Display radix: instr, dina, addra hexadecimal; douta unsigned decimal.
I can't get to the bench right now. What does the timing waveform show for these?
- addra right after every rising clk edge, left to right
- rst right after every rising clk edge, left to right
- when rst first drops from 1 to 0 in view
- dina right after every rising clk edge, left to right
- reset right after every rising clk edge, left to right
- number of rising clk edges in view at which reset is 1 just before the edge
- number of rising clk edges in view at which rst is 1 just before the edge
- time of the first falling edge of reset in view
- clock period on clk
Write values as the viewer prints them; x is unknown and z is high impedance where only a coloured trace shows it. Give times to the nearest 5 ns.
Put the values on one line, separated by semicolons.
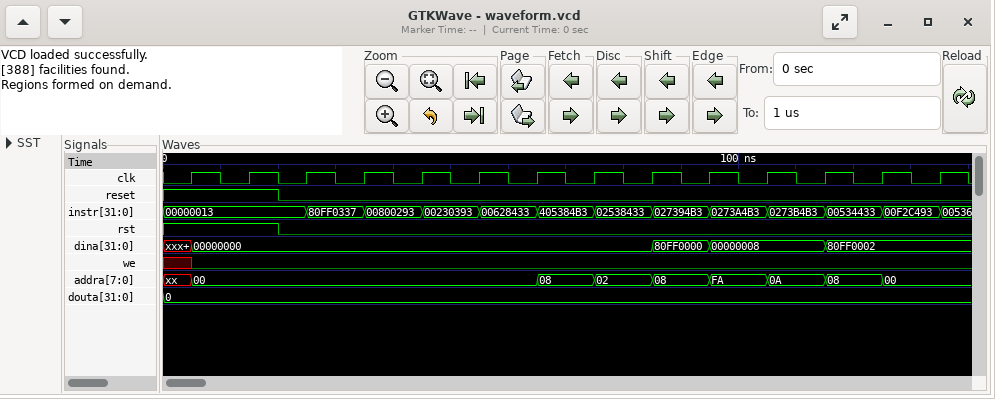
00, 00, 00, 00, 00, 00, 08, 02, 08, FA, 0A, 08, 00, 00; 1 1 0 0 0 0 0 0 0 0 0 0 0 0; 20 ns; 00000000, 00000000, 00000000, 00000000, 00000000, 00000000, 00000000, 00000000, 80FF0000, 00000008, 00000008, 80FF0002, 80FF0002, 80FF0002; 1 1 0 0 0 0 0 0 0 0 0 0 0 0; 2; 2; 20 ns; 10 ns
